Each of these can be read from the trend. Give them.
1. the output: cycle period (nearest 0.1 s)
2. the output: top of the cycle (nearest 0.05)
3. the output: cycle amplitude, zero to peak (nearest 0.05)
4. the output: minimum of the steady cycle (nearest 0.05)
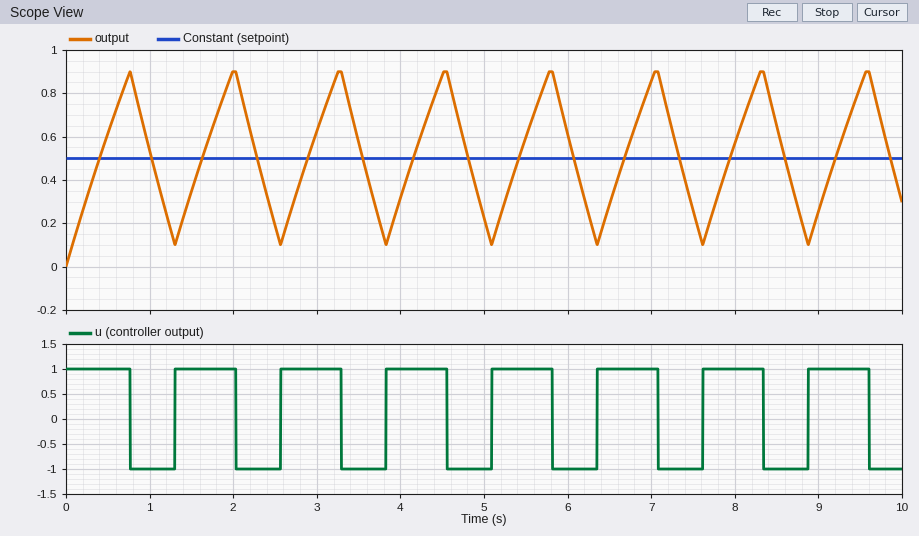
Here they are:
1.3 s
0.90
0.40
0.10
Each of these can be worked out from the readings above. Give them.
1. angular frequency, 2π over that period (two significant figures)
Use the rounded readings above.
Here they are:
4.8 rad/s
